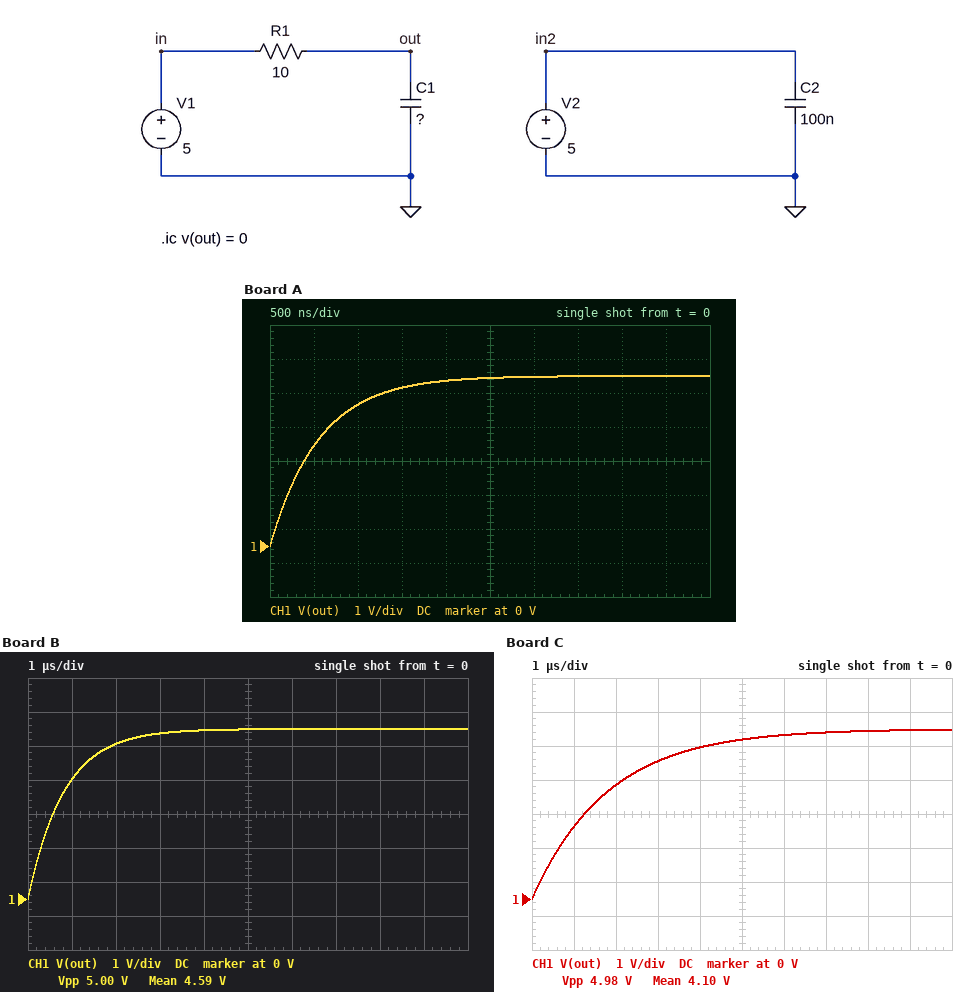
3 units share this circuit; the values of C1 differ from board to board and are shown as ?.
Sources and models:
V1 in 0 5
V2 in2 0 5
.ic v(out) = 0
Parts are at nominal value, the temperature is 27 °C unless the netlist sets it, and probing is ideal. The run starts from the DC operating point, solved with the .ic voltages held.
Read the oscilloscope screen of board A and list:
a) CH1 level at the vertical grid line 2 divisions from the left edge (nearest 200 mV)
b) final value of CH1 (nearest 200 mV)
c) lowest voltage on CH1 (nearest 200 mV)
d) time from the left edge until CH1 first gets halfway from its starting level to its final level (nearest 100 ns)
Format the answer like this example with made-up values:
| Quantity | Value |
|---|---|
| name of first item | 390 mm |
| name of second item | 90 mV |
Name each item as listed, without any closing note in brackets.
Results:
| Quantity | Value |
|---|---|
| CH1 level at the vertical grid line 2 divisions from the left edge | 4.2 V |
| final value of CH1 | 5.0 V |
| lowest voltage on CH1 | 0 V |
| time from the left edge until CH1 first gets halfway from its starting level to its final level | 400 ns |
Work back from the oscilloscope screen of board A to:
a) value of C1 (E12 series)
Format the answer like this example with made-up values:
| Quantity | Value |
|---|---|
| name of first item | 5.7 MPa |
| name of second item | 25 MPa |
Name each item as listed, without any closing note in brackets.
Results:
| Quantity | Value |
|---|---|
| value of C1 | 56 nF |
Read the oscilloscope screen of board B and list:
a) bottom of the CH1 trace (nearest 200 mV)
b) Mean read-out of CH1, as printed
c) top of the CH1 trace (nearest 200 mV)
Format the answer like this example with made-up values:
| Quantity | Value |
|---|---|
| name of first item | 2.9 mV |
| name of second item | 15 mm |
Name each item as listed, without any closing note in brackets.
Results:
| Quantity | Value |
|---|---|
| bottom of the CH1 trace | 0 V |
| Mean read-out of CH1, as printed | 4.59 V |
| top of the CH1 trace | 5.0 V |
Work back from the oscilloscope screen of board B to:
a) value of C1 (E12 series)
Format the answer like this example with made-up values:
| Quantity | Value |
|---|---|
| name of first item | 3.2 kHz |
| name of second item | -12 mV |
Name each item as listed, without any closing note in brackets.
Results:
| Quantity | Value |
|---|---|
| value of C1 | 82 nF |
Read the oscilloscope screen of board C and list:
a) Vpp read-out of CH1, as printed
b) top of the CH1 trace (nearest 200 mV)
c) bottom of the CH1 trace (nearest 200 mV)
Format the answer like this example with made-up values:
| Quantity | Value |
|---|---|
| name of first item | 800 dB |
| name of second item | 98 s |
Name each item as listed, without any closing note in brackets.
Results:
| Quantity | Value |
|---|---|
| Vpp read-out of CH1, as printed | 4.98 V |
| top of the CH1 trace | 5.0 V |
| bottom of the CH1 trace | 0 V |
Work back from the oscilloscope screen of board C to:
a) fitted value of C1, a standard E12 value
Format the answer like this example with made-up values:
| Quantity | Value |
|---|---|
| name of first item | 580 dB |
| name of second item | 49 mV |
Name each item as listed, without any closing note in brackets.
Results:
| Quantity | Value |
|---|---|
| fitted value of C1, a standard E12 value | 180 nF |
